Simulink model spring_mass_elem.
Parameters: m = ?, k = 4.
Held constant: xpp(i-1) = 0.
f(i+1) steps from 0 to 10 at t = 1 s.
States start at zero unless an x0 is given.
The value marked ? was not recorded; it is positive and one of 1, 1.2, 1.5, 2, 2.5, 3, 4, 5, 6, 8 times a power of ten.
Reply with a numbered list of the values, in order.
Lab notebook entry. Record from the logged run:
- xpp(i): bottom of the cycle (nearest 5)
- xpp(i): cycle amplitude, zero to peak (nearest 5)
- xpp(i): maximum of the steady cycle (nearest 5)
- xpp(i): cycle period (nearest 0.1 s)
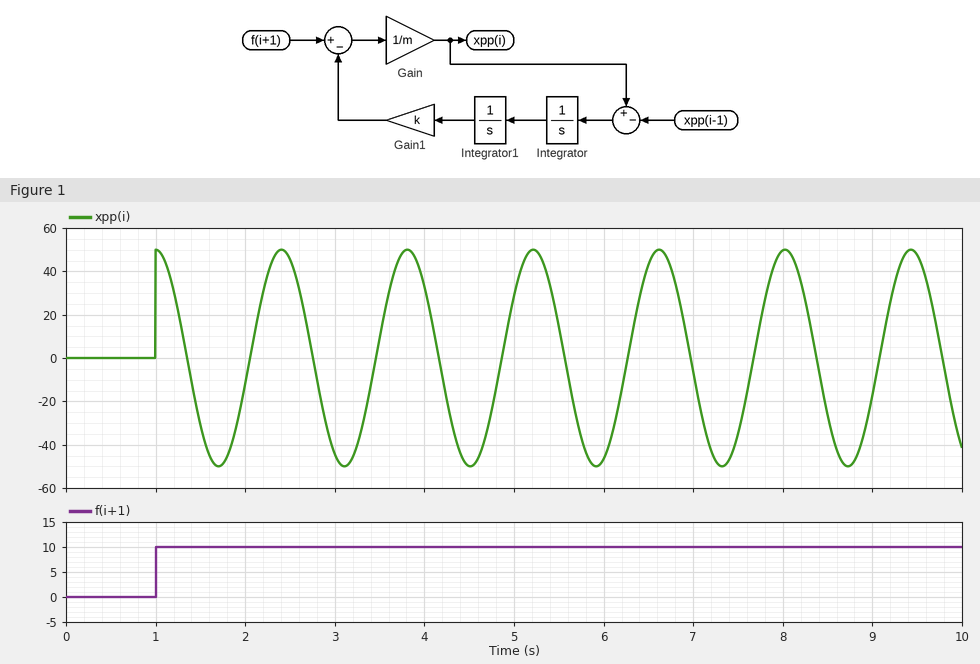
1. -50
2. 50
3. 50
4. 1.4 s
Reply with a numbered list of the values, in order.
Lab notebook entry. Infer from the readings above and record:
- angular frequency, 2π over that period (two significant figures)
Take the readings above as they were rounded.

1. 4.5 rad/s
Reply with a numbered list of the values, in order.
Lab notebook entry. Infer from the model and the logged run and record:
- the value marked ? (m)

1. 0.2
